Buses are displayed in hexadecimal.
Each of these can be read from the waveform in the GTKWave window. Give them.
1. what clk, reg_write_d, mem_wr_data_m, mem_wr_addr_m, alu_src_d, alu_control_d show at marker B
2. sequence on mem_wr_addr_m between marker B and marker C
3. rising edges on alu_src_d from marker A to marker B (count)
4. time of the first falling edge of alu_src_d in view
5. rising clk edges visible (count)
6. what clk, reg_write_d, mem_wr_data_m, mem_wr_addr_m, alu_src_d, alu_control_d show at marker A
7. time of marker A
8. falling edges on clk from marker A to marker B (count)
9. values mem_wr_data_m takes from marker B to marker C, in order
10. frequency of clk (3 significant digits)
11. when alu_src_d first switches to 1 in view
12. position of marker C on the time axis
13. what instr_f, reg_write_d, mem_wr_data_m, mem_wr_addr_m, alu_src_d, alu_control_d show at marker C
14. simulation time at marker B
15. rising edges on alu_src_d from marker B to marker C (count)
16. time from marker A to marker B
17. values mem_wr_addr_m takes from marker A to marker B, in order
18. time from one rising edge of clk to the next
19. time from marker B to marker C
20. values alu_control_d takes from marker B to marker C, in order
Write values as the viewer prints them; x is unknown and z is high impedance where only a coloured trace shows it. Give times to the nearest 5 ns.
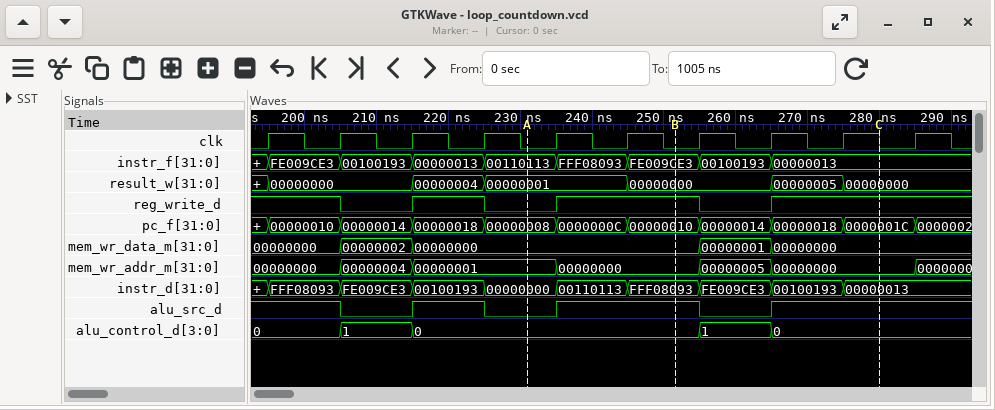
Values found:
clk=0, reg_write_d=1, mem_wr_data_m=00000000, mem_wr_addr_m=00000000, alu_src_d=1, alu_control_d=0
00000000, 00000005, 00000000
1
205 ns
10
clk=0, reg_write_d=0, mem_wr_data_m=00000000, mem_wr_addr_m=00000001, alu_src_d=0, alu_control_d=0
230 ns
2
00000000, 00000001, 00000000
100 MHz
215 ns
280 ns
instr_f=00000013, reg_write_d=1, mem_wr_data_m=00000000, mem_wr_addr_m=00000000, alu_src_d=1, alu_control_d=0
250 ns
1
20 ns
00000001, 00000000
10 ns
30 ns
0, 1, 0
